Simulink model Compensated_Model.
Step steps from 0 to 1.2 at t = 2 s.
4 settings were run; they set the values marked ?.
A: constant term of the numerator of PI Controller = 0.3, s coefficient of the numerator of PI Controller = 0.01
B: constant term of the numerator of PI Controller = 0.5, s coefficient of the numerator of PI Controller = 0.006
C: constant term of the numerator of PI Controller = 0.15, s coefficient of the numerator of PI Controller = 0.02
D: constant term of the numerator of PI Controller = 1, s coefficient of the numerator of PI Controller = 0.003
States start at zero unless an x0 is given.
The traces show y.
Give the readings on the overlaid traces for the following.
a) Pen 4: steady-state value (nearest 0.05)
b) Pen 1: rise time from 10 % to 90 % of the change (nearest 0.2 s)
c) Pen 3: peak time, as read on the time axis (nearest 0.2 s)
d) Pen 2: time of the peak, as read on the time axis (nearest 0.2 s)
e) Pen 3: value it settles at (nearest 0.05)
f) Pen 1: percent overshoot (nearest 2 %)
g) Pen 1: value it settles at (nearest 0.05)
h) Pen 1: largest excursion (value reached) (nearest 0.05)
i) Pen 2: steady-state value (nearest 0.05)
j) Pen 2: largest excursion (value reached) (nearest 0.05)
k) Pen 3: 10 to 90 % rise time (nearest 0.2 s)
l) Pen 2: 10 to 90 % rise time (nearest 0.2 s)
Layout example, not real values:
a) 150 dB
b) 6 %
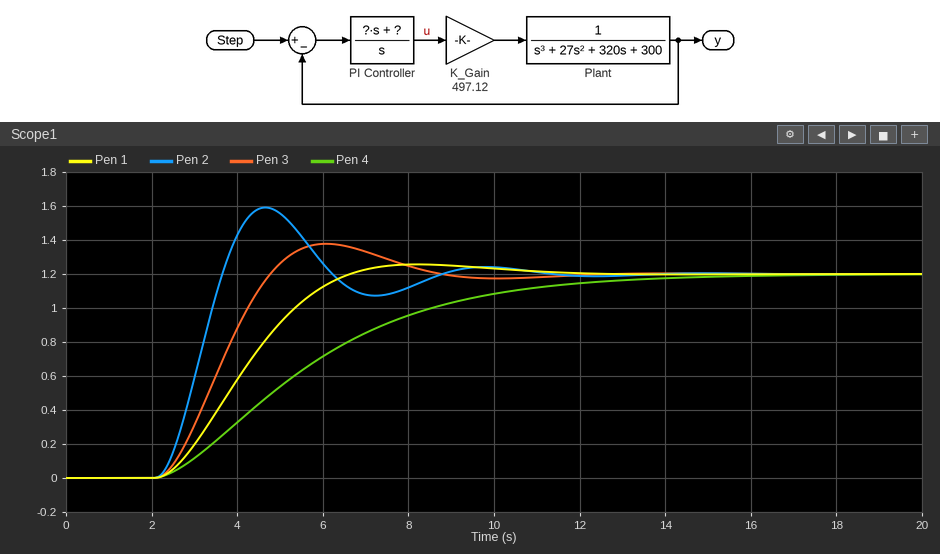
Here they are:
a) 1.20
b) 3.0 s
c) 6.0 s
d) 4.6 s
e) 1.20
f) 4 %
g) 1.20
h) 1.25
i) 1.20
j) 1.60
k) 1.8 s
l) 1.0 s
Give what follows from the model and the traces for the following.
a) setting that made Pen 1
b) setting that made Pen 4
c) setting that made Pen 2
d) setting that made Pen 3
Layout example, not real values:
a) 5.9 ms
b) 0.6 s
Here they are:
a) A
b) C
c) D
d) B
